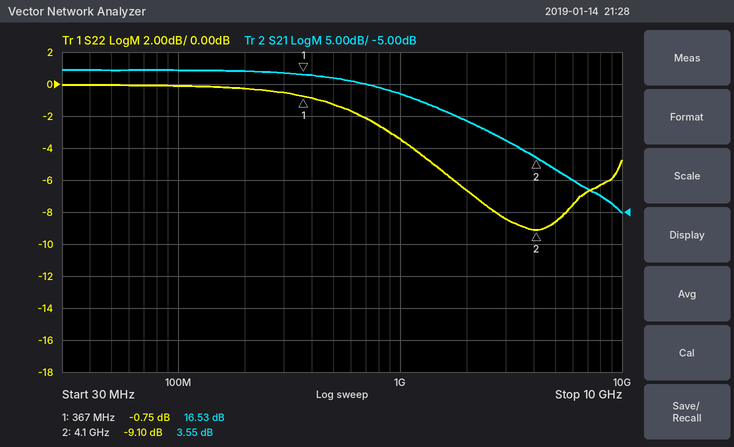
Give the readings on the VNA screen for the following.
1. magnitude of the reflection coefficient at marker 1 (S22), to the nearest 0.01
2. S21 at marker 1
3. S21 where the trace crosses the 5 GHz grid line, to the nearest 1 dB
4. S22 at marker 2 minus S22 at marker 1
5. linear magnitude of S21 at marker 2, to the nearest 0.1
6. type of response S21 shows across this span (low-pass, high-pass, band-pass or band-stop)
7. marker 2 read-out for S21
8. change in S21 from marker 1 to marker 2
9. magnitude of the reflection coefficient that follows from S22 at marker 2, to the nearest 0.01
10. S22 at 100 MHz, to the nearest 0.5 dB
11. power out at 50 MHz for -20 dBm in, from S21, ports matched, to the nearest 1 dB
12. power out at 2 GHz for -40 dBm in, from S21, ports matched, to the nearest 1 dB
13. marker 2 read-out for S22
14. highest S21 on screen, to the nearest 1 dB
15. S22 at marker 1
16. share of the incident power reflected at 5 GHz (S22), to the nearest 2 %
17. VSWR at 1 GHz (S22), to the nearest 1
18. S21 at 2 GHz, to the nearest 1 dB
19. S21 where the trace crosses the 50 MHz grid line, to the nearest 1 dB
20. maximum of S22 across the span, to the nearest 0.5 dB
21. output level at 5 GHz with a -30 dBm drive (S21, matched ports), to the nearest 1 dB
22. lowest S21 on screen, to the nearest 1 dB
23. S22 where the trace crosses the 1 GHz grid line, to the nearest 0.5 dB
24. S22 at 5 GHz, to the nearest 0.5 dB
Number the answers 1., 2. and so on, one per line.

1. 0.92
2. 16.53 dB
3. 2 dB
4. -8.35 dB
5. 1.5
6. low-pass
7. 3.55 dB
8. -12.98 dB
9. 0.35
10. 0.0 dB
11. -3 dBm
12. -31 dBm
13. -9.10 dB
14. 17 dB
15. -0.75 dB
16. 14 %
17. 5
18. 9 dB
19. 17 dB
20. 0.0 dB
21. -28 dBm
22. -5 dB
23. -3.5 dB
24. -8.5 dB
